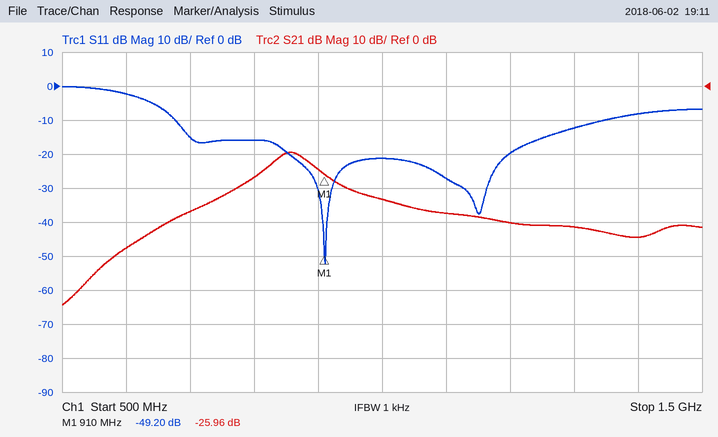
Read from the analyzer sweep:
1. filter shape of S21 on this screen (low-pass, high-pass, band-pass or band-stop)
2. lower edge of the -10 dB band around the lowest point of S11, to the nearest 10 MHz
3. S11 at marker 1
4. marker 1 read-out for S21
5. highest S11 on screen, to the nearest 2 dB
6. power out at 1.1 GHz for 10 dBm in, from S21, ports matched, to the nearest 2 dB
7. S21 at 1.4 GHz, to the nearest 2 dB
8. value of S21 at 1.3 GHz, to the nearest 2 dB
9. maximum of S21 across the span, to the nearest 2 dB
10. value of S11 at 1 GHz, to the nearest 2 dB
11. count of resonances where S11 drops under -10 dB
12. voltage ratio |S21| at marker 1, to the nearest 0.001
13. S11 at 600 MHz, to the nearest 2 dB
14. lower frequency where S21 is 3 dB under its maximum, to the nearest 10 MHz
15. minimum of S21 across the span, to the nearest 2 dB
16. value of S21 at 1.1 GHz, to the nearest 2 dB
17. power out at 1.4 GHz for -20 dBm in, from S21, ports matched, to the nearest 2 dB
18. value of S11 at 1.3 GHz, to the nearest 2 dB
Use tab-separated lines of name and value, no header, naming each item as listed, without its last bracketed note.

filter shape of S21 on this screen	band-pass
lower edge of the -10 dB band around the lowest point of S11, to the nearest 10 MHz	680 MHz
S11 at marker 1	-49.20 dB
marker 1 read-out for S21	-25.96 dB
highest S11 on screen, to the nearest 2 dB	0 dB
power out at 1.1 GHz for 10 dBm in, from S21, ports matched, to the nearest 2 dB	-28 dBm
S21 at 1.4 GHz, to the nearest 2 dB	-44 dB
value of S21 at 1.3 GHz, to the nearest 2 dB	-42 dB
maximum of S21 across the span, to the nearest 2 dB	-20 dB
value of S11 at 1 GHz, to the nearest 2 dB	-22 dB
count of resonances where S11 drops under -10 dB	2
voltage ratio |S21| at marker 1, to the nearest 0.001	0.050
S11 at 600 MHz, to the nearest 2 dB	-2 dB
lower frequency where S21 is 3 dB under its maximum, to the nearest 10 MHz	830 MHz
minimum of S21 across the span, to the nearest 2 dB	-64 dB
value of S21 at 1.1 GHz, to the nearest 2 dB	-38 dB
power out at 1.4 GHz for -20 dBm in, from S21, ports matched, to the nearest 2 dB	-64 dBm
value of S11 at 1.3 GHz, to the nearest 2 dB	-12 dB
